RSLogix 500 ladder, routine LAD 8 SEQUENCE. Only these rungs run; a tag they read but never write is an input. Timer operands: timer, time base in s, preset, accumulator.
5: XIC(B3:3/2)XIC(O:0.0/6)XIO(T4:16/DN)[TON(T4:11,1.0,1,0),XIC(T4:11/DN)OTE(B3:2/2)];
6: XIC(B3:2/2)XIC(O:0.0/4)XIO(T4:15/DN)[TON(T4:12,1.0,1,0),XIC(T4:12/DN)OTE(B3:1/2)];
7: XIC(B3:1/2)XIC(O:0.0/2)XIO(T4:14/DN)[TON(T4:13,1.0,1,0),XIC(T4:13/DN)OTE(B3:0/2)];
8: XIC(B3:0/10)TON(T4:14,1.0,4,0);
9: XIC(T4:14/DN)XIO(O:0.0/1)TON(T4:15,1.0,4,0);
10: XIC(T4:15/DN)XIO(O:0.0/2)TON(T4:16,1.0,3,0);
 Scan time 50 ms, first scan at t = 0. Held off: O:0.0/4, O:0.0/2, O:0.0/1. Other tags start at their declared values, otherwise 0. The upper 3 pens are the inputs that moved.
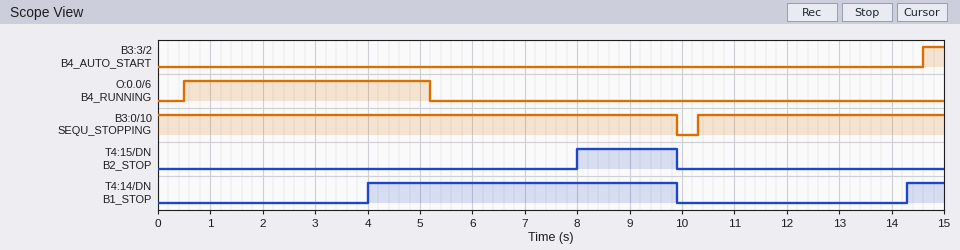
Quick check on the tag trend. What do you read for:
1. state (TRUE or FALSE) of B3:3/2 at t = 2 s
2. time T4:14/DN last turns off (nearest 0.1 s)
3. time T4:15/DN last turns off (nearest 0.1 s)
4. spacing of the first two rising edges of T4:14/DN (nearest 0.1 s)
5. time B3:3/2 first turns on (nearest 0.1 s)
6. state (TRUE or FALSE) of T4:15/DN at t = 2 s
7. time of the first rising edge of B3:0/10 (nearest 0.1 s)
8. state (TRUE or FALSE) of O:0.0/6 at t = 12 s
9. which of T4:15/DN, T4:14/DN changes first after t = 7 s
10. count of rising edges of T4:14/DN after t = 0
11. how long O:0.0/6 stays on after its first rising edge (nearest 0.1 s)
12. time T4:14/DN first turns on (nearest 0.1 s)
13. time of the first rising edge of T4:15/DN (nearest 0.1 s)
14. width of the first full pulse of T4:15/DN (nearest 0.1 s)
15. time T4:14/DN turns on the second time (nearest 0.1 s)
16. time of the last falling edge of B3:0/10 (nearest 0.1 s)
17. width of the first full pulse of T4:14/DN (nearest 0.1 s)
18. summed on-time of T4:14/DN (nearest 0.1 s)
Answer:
FALSE
9.9 s
9.9 s
10.3 s
14.6 s
FALSE
10.3 s
FALSE
T4:15/DN
2
4.7 s
4.0 s
8.0 s
1.9 s
14.3 s
9.9 s
5.9 s
6.6 s
